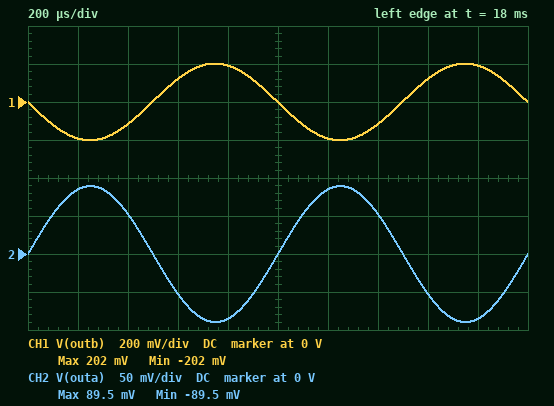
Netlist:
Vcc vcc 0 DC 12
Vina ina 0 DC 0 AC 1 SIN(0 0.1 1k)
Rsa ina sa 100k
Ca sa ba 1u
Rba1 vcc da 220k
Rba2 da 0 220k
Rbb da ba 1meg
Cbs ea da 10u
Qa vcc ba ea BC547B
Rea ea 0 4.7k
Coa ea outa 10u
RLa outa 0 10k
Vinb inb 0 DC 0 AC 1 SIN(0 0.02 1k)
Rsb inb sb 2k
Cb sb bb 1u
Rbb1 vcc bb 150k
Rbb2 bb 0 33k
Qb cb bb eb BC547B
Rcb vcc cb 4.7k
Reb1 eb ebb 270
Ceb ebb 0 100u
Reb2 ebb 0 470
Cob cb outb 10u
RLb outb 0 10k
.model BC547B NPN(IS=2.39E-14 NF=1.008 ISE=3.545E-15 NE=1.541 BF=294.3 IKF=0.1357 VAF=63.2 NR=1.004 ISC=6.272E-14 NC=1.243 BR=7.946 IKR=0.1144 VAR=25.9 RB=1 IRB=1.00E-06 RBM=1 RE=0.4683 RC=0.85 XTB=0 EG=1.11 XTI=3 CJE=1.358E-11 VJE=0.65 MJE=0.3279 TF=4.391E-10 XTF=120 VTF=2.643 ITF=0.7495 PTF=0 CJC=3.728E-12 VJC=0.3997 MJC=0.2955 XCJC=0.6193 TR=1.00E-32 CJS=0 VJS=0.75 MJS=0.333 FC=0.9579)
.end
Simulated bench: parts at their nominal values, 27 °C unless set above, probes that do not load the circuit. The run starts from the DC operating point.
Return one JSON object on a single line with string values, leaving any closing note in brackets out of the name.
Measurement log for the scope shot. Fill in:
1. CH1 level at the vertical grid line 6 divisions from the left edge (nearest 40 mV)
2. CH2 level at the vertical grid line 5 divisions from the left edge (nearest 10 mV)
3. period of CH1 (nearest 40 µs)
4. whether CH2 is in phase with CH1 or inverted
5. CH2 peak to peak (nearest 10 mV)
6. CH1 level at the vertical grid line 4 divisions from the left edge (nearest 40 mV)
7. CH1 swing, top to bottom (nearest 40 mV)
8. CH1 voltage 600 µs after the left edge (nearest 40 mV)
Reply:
{"CH1 level at the vertical grid line 6 divisions from the left edge": "-200 mV", "CH2 level at the vertical grid line 5 divisions from the left edge": "0 V", "period of CH1": "1.00 ms", "whether CH2 is in phase with CH1 or inverted": "inverted", "CH2 peak to peak": "180 mV", "CH1 level at the vertical grid line 4 divisions from the left edge": "200 mV", "CH1 swing, top to bottom": "400 mV", "CH1 voltage 600 µs after the left edge": "120 mV"}
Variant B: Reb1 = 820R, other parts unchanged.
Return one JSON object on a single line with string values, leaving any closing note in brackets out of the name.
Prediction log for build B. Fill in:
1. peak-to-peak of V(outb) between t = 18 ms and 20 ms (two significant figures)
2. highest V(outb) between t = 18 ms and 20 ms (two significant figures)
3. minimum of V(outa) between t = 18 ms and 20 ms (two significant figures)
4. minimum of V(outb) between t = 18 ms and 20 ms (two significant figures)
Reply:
{"peak-to-peak of V(outb) between t = 18 ms and 20 ms": "140 mV", "highest V(outb) between t = 18 ms and 20 ms": "70 mV", "minimum of V(outa) between t = 18 ms and 20 ms": "-90 mV", "minimum of V(outb) between t = 18 ms and 20 ms": "-69 mV"}
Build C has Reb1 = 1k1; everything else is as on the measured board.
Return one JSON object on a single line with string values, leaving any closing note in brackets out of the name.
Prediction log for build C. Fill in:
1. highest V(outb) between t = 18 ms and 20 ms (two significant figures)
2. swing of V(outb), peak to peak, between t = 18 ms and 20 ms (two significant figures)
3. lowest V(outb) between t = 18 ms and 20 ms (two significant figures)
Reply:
{"highest V(outb) between t = 18 ms and 20 ms": "52 mV", "swing of V(outb), peak to peak, between t = 18 ms and 20 ms": "100 mV", "lowest V(outb) between t = 18 ms and 20 ms": "-52 mV"}
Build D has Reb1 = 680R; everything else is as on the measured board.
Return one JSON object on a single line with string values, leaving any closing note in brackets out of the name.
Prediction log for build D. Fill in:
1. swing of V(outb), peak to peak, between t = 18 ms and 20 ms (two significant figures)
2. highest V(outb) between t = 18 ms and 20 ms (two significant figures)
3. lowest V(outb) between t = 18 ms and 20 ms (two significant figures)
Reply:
{"swing of V(outb), peak to peak, between t = 18 ms and 20 ms": "170 mV", "highest V(outb) between t = 18 ms and 20 ms": "84 mV", "lowest V(outb) between t = 18 ms and 20 ms": "-83 mV"}
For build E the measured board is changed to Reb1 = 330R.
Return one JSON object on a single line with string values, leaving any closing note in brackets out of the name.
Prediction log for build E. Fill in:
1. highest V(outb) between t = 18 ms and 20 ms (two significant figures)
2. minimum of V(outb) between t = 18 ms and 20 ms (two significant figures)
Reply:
{"highest V(outb) between t = 18 ms and 20 ms": "170 mV", "minimum of V(outb) between t = 18 ms and 20 ms": "-170 mV"}
